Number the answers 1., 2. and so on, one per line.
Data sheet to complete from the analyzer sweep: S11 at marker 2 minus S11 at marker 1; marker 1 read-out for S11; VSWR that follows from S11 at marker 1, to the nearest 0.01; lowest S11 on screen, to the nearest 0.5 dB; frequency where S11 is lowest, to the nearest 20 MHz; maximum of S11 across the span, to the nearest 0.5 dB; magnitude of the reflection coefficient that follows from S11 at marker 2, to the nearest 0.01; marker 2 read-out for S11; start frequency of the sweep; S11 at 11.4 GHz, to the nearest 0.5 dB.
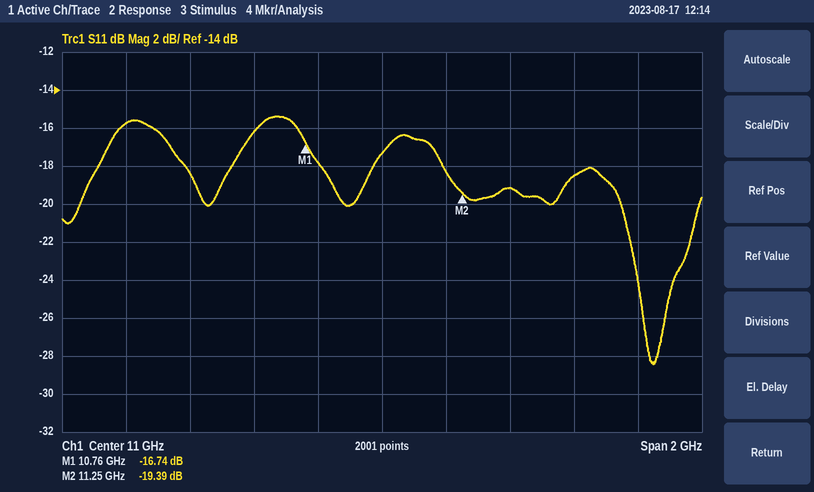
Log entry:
1. -2.65 dB
2. -16.74 dB
3. 1.34
4. -28.5 dB
5. 11.84 GHz
6. -15.5 dB
7. 0.11
8. -19.39 dB
9. 10 GHz
10. -19.0 dB
